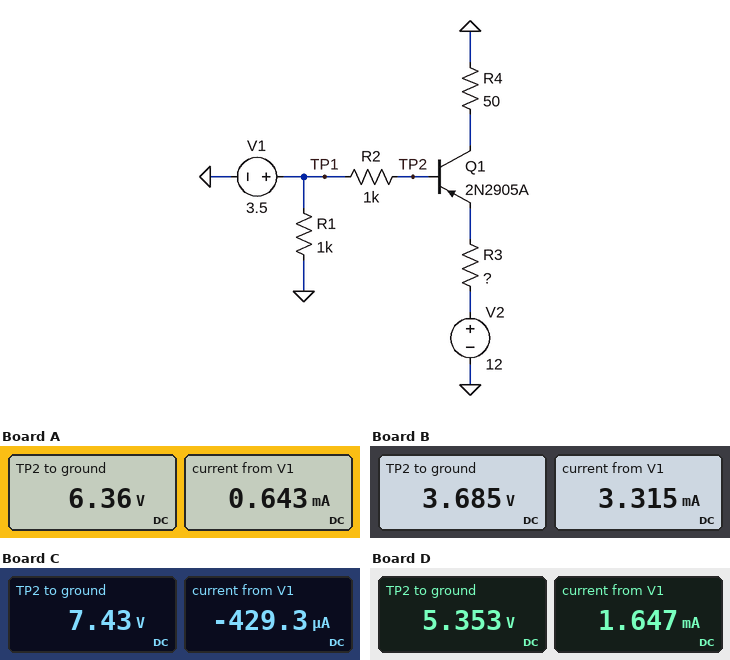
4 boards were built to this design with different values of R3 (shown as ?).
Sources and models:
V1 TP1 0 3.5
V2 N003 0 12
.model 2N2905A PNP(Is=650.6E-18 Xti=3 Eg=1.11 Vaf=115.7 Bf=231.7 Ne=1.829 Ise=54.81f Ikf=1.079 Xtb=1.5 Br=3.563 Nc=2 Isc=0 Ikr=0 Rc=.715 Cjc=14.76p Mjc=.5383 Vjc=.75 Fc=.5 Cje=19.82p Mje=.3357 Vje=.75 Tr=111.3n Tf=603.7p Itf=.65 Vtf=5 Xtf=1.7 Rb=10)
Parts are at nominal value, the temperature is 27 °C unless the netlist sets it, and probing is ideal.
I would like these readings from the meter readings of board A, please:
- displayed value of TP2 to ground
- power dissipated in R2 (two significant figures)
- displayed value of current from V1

6.36 V
8.2 mW
0.643 mA
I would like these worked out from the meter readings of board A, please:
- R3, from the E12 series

33 Ω
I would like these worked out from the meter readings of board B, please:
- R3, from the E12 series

180 Ω
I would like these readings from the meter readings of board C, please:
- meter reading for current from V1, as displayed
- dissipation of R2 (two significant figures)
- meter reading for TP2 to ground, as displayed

-429.3 µA
15 mW
7.43 V
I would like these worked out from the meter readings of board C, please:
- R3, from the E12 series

22 Ω
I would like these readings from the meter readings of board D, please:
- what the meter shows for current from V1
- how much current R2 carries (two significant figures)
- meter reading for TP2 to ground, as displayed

1.647 mA
1.9 mA
5.353 V
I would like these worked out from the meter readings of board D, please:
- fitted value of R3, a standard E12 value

47 Ω
